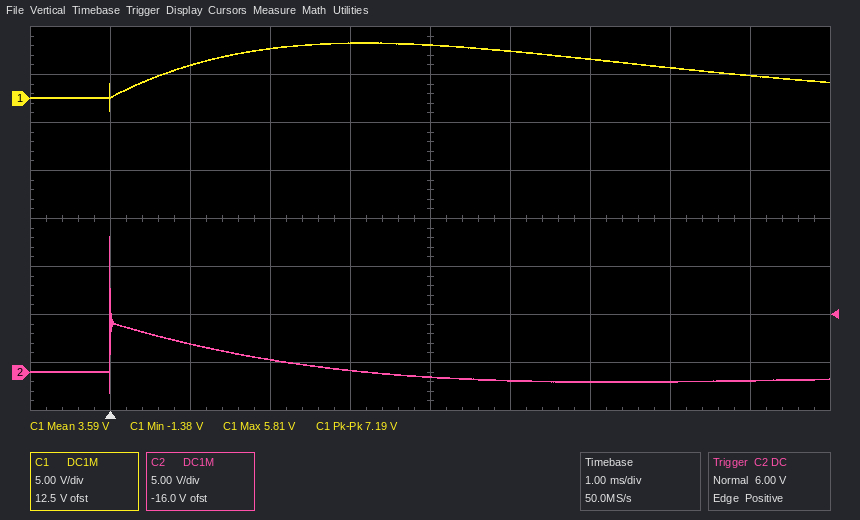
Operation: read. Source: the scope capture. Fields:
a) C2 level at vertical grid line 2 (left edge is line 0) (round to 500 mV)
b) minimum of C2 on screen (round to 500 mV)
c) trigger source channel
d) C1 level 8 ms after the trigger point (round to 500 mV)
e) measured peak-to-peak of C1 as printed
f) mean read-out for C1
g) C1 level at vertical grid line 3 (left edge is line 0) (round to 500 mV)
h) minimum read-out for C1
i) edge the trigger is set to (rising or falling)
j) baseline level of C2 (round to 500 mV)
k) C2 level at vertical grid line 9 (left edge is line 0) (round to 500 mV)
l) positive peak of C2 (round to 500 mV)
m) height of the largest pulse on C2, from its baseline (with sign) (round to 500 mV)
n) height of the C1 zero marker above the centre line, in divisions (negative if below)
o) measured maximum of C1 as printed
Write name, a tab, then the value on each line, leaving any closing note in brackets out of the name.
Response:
C2 level at vertical grid line 2 (left edge is line 0)	3.0 V
minimum of C2 on screen	-2.0 V
trigger source channel	C2
C1 level 8 ms after the trigger point	2.5 V
measured peak-to-peak of C1 as printed	7.19 V
mean read-out for C1	3.59 V
C1 level at vertical grid line 3 (left edge is line 0)	5.0 V
minimum read-out for C1	-1.38 V
edge the trigger is set to	rising
baseline level of C2	-1.0 V
C2 level at vertical grid line 9 (left edge is line 0)	-1.0 V
positive peak of C2	14.0 V
height of the largest pulse on C2, from its baseline (with sign)	+15.0 V
height of the C1 zero marker above the centre line, in divisions	+2.5 div
measured maximum of C1 as printed	5.81 V
